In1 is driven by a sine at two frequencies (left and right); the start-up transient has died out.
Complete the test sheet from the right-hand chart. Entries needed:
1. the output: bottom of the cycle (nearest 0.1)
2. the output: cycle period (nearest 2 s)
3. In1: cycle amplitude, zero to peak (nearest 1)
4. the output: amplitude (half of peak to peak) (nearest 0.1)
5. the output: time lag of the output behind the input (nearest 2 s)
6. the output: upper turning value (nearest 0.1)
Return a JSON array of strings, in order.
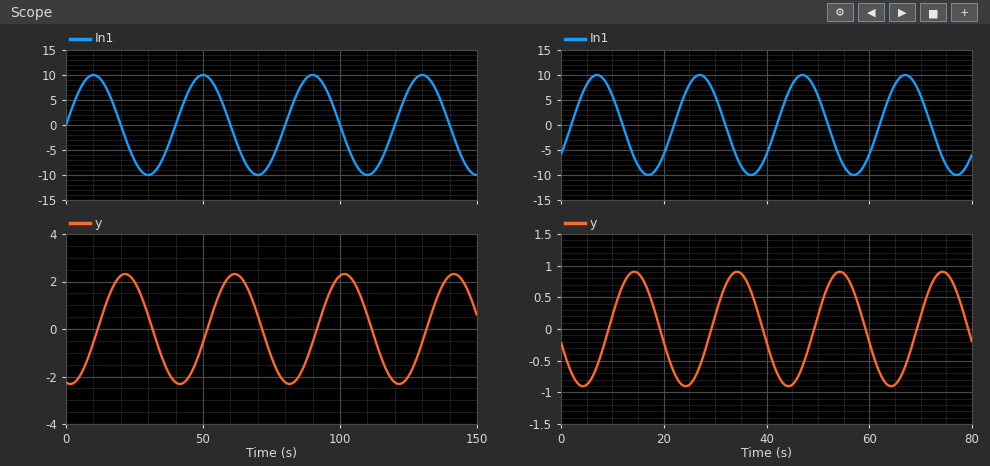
["-0.9", "20 s", "10", "0.9", "8 s", "0.9"]
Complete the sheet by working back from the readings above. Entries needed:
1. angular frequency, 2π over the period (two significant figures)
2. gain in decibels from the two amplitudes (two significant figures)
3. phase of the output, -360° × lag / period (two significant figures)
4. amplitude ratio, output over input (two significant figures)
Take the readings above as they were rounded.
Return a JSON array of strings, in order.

["0.31 rad/s", "-21 dB", "-140°", "0.090"]
